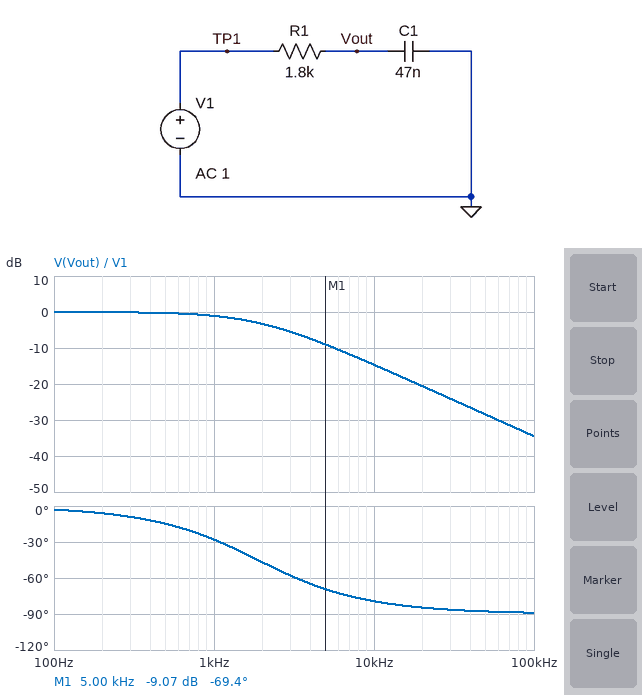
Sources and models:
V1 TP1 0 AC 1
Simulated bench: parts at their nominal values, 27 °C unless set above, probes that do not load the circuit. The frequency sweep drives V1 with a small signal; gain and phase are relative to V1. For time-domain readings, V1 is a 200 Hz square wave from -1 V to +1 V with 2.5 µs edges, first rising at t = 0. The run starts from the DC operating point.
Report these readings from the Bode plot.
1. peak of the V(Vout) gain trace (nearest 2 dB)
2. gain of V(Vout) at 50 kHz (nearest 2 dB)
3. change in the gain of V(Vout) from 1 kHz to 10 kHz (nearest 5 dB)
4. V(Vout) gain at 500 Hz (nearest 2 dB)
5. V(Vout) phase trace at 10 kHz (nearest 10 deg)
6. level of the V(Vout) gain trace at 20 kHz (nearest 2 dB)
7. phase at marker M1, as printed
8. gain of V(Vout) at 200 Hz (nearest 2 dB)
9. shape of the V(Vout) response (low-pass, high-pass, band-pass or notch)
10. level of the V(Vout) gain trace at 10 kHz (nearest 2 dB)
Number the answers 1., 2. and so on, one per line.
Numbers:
1. 0 dB
2. -28 dB
3. -15 dB
4. 0 dB
5. -80 deg
6. -20 dB
7. -69.4 deg
8. 0 dB
9. low-pass
10. -14 dB
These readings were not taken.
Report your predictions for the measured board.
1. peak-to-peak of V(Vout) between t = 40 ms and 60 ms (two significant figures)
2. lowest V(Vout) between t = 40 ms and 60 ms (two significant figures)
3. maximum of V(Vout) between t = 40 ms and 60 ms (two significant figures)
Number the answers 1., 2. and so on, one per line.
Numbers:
1. 2.0 V
2. -1.0 V
3. 1.0 V
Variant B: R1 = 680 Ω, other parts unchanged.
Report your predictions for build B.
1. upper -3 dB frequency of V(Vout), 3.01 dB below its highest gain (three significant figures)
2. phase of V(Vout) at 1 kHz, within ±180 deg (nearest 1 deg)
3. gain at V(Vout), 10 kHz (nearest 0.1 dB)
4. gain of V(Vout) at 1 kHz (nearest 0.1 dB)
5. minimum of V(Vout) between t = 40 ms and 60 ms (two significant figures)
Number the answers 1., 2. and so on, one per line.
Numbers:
1. 4.98 kHz
2. -11 deg
3. -7.0 dB
4. -0.2 dB
5. -1.0 V
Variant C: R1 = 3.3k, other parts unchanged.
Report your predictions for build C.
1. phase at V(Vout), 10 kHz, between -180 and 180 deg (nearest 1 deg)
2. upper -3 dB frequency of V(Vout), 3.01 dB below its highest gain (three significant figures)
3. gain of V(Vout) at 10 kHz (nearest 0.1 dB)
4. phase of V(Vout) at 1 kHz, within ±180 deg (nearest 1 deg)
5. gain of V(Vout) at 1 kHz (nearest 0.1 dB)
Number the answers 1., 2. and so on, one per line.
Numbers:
1. -84 deg
2. 1.03 kHz
3. -19.8 dB
4. -44 deg
5. -2.9 dB
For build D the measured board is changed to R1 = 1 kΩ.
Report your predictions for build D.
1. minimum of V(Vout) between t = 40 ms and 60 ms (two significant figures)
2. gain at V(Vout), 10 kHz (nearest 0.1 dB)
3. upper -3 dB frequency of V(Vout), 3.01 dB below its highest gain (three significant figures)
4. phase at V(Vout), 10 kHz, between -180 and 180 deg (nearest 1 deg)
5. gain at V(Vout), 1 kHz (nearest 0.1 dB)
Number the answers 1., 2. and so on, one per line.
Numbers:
1. -1.0 V
2. -9.9 dB
3. 3.39 kHz
4. -71 deg
5. -0.4 dB
